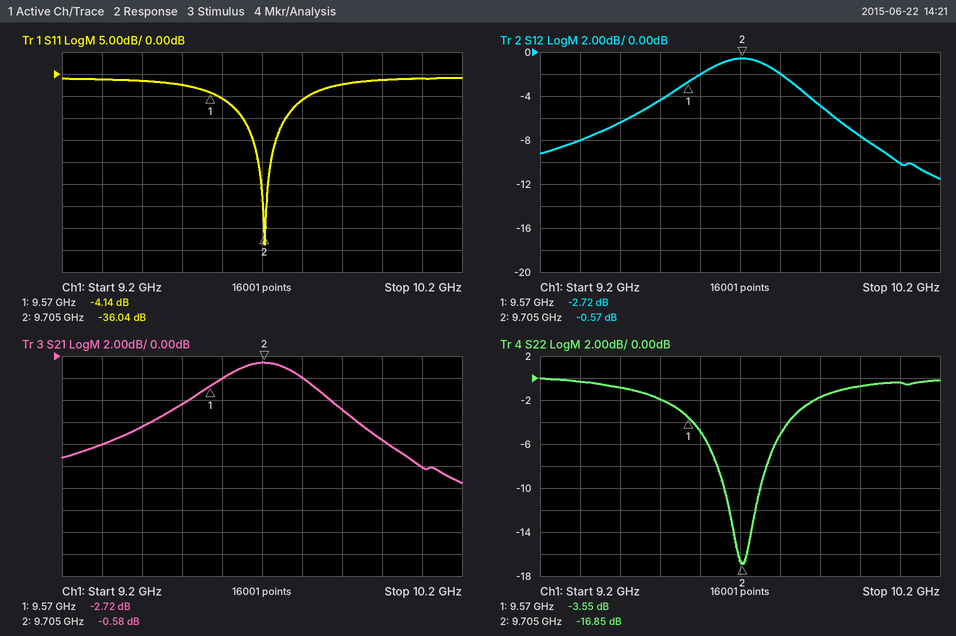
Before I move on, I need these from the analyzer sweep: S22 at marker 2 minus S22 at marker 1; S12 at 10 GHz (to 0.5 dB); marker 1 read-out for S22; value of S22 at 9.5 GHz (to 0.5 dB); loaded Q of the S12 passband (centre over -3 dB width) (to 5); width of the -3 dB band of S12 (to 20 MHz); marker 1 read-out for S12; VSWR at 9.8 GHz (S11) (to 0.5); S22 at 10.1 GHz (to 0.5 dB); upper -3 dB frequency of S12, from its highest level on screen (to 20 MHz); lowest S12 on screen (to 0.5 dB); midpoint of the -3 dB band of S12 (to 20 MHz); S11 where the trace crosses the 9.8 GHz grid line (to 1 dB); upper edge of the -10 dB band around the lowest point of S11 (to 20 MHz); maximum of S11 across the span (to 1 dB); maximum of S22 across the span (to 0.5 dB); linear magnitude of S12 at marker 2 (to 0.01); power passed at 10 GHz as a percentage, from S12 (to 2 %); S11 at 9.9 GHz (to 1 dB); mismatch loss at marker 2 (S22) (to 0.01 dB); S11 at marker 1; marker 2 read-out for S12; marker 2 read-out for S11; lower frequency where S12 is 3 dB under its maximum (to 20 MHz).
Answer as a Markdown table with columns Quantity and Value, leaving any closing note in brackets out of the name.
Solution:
| Quantity | Value |
|---|---|
| S22 at marker 2 minus S22 at marker 1 | -13.30 dB |
| S12 at 10 GHz | -7.5 dB |
| marker 1 read-out for S22 | -3.55 dB |
| value of S22 at 9.5 GHz | -2.0 dB |
| loaded Q of the S12 passband (centre over -3 dB width) | 30 |
| width of the -3 dB band of S12 | 320 MHz |
| marker 1 read-out for S12 | -2.72 dB |
| VSWR at 9.8 GHz (S11) | 3.0 |
| S22 at 10.1 GHz | -0.5 dB |
| upper -3 dB frequency of S12, from its highest level on screen | 9.86 GHz |
| lowest S12 on screen | -11.5 dB |
| midpoint of the -3 dB band of S12 | 9.70 GHz |
| S11 where the trace crosses the 9.8 GHz grid line | -6 dB |
| upper edge of the -10 dB band around the lowest point of S11 | 9.76 GHz |
| maximum of S11 across the span | -1 dB |
| maximum of S22 across the span | 0.0 dB |
| linear magnitude of S12 at marker 2 | 0.94 |
| power passed at 10 GHz as a percentage, from S12 | 18 % |
| S11 at 9.9 GHz | -2 dB |
| mismatch loss at marker 2 (S22) | 0.09 dB |
| S11 at marker 1 | -4.14 dB |
| marker 2 read-out for S12 | -0.57 dB |
| marker 2 read-out for S11 | -36.04 dB |
| lower frequency where S12 is 3 dB under its maximum | 9.54 GHz |
